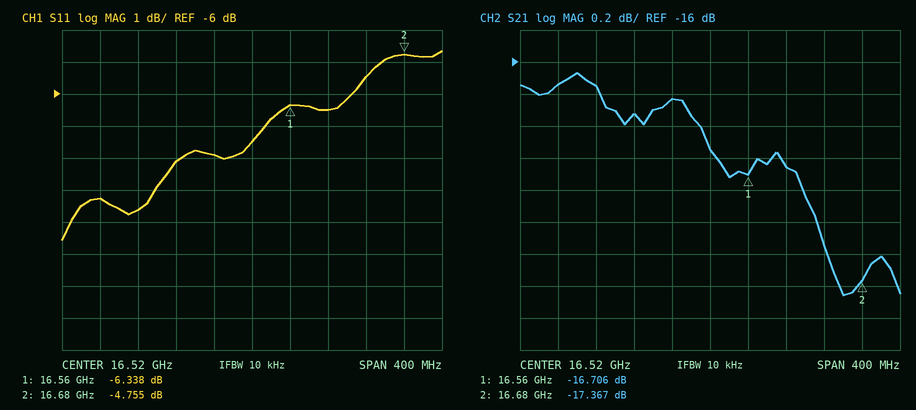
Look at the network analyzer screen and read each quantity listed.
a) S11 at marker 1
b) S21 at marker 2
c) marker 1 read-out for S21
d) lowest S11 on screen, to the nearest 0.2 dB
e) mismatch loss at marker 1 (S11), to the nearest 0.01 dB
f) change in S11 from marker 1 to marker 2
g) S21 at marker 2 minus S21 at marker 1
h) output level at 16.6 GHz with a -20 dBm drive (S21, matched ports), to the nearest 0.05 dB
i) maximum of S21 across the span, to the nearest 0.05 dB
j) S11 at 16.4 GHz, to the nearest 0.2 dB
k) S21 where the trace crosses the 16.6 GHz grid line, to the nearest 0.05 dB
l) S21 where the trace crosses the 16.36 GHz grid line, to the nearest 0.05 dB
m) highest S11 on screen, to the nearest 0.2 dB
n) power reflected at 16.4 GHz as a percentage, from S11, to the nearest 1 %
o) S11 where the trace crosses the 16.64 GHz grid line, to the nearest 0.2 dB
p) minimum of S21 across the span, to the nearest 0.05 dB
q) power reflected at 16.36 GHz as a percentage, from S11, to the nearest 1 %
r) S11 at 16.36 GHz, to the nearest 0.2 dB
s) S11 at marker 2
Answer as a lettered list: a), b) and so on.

a) -6.338 dB
b) -17.367 dB
c) -16.706 dB
d) -10.6 dB
e) 1.15 dB
f) 1.583 dB
g) -0.661 dB
h) -36.65 dBm
i) -16.05 dB
j) -9.6 dB
k) -16.65 dB
l) -16.15 dB
m) -4.6 dB
n) 11 %
o) -5.4 dB
p) -17.45 dB
q) 12 %
r) -9.2 dB
s) -4.755 dB
